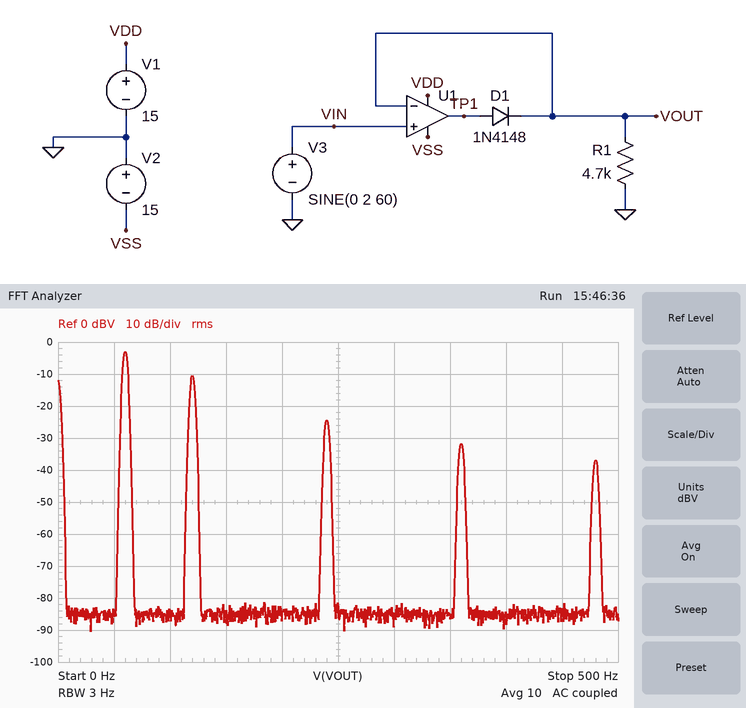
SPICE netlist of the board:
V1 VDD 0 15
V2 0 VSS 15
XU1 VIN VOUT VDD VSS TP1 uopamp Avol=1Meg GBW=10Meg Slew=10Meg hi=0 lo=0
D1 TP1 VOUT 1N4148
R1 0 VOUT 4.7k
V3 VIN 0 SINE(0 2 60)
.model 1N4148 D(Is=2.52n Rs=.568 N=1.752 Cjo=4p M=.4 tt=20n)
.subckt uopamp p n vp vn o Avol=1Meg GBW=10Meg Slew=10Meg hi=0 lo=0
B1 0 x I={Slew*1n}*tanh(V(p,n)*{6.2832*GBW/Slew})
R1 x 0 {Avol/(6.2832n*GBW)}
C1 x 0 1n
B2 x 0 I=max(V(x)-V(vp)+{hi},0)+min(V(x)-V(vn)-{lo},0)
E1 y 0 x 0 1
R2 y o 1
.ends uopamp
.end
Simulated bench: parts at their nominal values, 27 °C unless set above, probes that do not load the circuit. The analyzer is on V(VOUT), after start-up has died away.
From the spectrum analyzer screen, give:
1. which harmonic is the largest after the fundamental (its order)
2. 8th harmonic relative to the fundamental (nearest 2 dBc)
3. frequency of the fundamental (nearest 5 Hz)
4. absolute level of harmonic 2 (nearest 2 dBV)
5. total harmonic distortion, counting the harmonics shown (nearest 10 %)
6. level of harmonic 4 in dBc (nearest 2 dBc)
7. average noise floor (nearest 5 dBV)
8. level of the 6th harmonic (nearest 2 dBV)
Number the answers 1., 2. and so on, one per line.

1. 2
2. -34 dBc
3. 60 Hz
4. -10 dBV
5. 40 %
6. -22 dBc
7. -85 dBV
8. -32 dBV
